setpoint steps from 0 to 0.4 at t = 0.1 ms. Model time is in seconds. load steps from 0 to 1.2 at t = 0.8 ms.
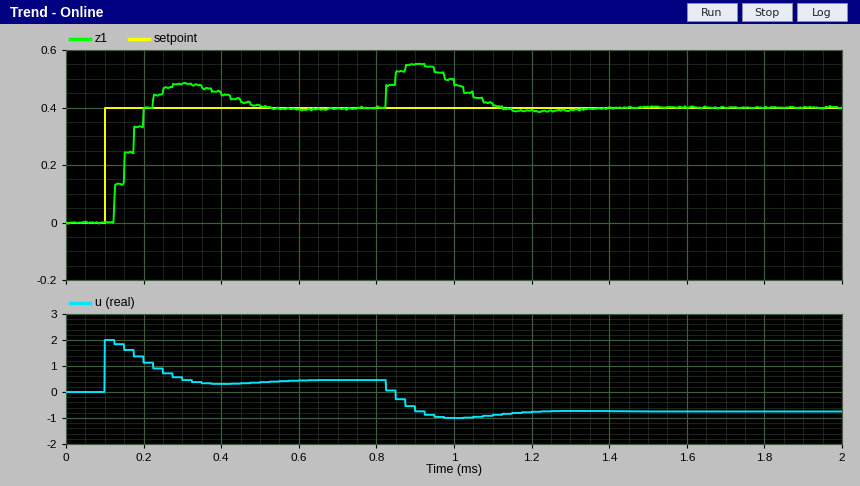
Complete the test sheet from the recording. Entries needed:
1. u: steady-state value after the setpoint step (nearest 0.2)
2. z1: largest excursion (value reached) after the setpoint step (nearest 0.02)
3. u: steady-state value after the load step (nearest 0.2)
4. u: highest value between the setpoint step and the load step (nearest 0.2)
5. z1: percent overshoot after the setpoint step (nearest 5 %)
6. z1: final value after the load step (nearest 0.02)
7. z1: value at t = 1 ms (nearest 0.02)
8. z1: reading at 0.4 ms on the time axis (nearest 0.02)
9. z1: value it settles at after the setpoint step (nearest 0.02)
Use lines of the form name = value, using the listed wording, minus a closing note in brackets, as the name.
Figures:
u: steady-state value after the setpoint step = 0.4
z1: largest excursion (value reached) after the setpoint step = 0.48
u: steady-state value after the load step = -0.8
u: highest value between the setpoint step and the load step = 2.0
z1: percent overshoot after the setpoint step = 20 %
z1: final value after the load step = 0.40
z1: value at t = 1 ms = 0.48
z1: reading at 0.4 ms on the time axis = 0.44
z1: value it settles at after the setpoint step = 0.40
